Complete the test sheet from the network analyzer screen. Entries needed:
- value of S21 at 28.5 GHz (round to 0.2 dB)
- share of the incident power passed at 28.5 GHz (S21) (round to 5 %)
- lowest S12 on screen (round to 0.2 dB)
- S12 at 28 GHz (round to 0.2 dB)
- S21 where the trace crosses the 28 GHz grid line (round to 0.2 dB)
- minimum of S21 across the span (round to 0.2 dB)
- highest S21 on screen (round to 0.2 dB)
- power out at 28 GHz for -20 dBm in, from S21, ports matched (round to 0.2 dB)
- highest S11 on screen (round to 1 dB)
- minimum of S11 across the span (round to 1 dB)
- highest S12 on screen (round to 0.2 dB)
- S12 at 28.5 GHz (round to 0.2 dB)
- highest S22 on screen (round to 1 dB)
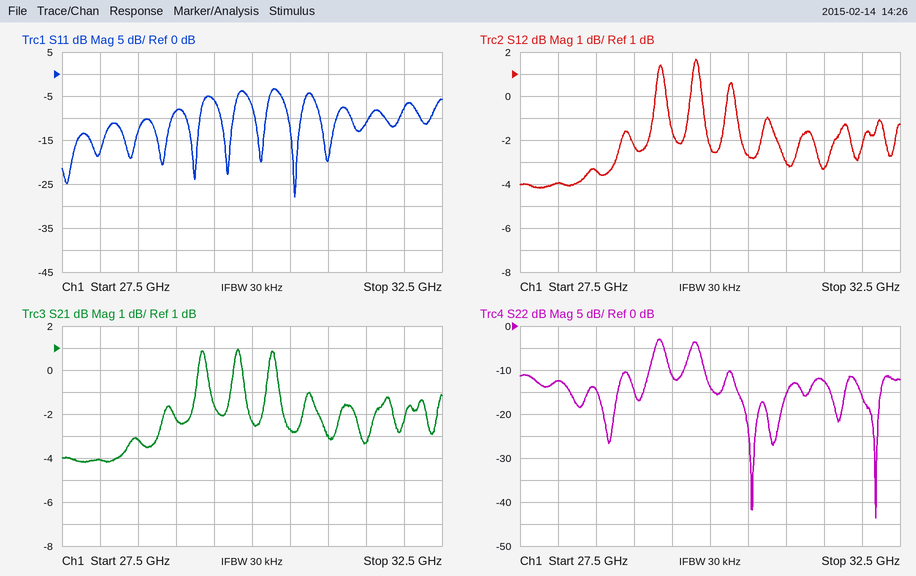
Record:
-3.2 dB
50 %
-4.2 dB
-4.0 dB
-4.0 dB
-4.2 dB
1.0 dB
-24.0 dBm
-3 dB
-28 dB
1.6 dB
-3.4 dB
-3 dB
